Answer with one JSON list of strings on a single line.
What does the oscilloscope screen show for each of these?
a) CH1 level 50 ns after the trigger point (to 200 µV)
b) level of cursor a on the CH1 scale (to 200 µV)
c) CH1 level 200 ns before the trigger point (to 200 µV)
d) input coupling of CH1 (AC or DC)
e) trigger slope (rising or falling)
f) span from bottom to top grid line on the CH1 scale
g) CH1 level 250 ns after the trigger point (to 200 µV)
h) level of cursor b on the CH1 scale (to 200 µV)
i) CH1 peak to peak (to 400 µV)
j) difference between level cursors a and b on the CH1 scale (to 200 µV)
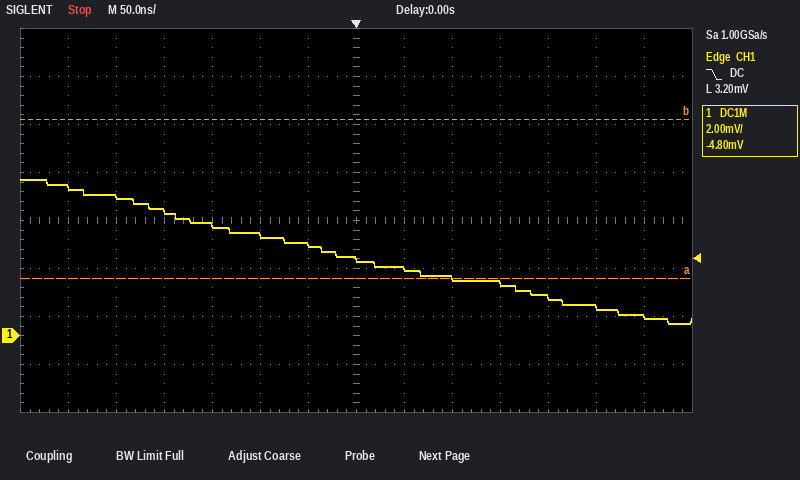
["2.8 mV", "2.4 mV", "5.2 mV", "DC", "falling", "16 mV", "1.2 mV", "9.0 mV", "6.0 mV", "6.6 mV"]
